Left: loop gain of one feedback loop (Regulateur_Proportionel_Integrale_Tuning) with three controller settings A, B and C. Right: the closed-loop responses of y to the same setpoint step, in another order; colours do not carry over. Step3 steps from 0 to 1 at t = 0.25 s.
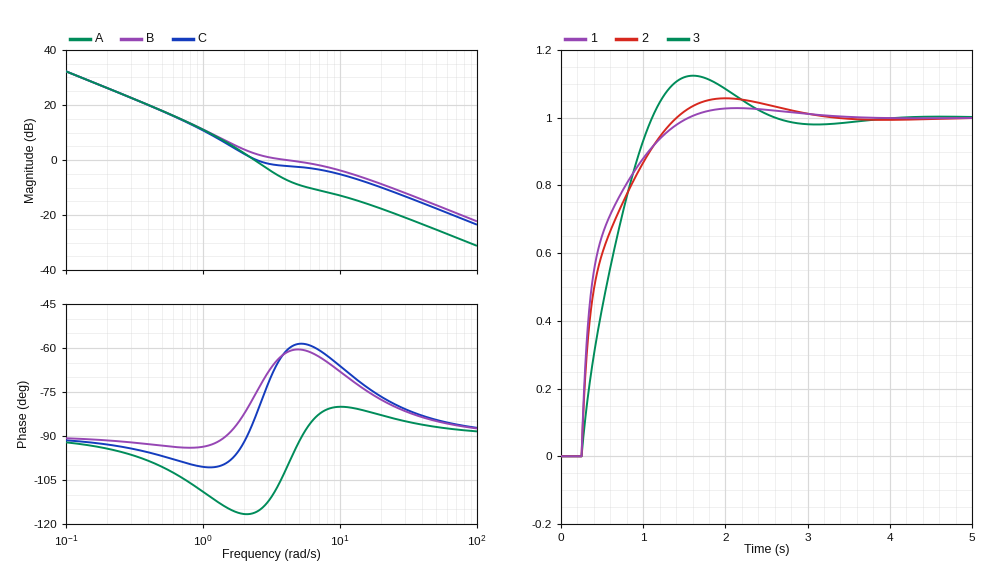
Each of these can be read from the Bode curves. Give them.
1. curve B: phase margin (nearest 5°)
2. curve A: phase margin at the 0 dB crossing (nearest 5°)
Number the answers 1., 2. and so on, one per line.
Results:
1. 120°
2. 65°
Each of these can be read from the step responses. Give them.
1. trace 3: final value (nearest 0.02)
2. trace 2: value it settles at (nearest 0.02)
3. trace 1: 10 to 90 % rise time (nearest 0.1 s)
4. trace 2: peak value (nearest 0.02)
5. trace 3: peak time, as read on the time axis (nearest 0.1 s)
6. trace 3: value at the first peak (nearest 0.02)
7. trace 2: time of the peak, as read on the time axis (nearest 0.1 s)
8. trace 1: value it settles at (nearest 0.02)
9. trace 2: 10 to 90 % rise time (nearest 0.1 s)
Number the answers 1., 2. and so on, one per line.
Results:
1. 1.00
2. 1.00
3. 0.8 s
4. 1.06
5. 1.6 s
6. 1.12
7. 2.0 s
8. 1.00
9. 0.8 s
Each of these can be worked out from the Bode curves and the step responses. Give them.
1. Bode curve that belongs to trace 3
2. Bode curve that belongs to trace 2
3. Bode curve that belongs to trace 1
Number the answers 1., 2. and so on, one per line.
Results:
1. A
2. C
3. B
